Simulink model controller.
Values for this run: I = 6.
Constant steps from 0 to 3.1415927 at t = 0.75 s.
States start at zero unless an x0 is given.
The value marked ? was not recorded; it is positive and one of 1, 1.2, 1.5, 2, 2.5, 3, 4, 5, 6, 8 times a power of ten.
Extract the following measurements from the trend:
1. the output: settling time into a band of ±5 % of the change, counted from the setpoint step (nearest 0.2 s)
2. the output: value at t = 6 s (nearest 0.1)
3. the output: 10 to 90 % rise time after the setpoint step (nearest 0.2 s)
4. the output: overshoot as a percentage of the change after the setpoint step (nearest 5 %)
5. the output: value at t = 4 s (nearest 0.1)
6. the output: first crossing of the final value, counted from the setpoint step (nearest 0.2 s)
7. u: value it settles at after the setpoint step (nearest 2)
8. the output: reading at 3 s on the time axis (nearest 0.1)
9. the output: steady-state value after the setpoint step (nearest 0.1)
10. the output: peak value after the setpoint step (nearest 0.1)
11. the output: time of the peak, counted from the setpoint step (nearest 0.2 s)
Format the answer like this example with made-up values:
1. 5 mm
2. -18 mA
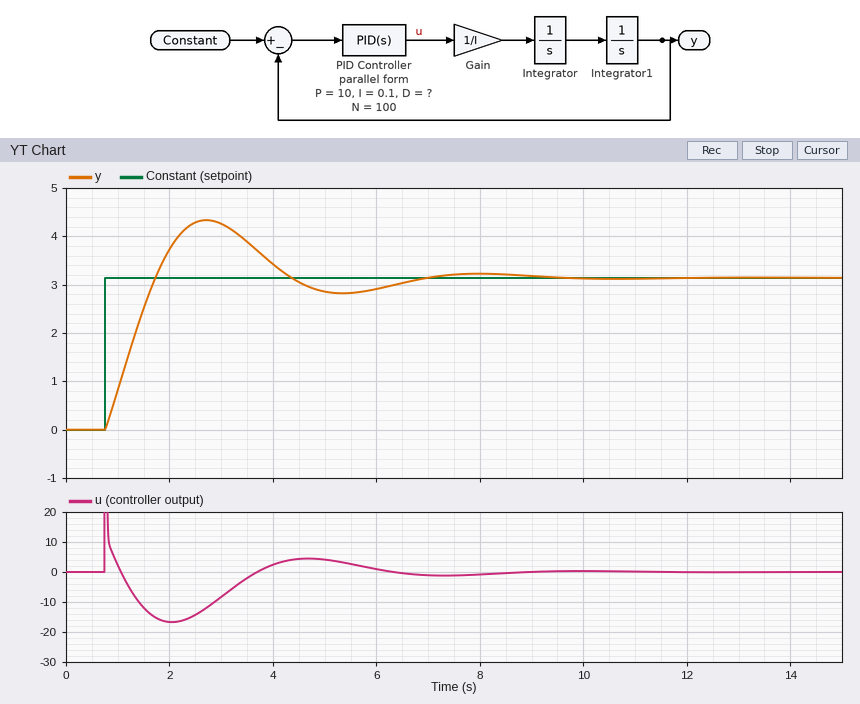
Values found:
1. 5.6 s
2. 2.9
3. 0.8 s
4. 40 %
5. 3.4
6. 1.0 s
7. 0
8. 4.3
9. 3.1
10. 4.3
11. 2.0 s
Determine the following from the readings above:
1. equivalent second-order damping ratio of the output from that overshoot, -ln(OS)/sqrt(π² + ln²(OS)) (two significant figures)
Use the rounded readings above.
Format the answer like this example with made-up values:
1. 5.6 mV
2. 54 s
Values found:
1. 0.28
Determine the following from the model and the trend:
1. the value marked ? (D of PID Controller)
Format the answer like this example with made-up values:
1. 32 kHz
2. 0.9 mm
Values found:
1. 6
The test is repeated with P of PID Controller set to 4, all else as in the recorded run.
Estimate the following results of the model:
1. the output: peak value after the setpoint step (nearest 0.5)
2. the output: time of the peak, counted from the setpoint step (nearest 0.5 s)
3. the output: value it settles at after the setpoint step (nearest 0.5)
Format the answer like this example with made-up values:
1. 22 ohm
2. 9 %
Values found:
1. 4.0
2. 3.0 s
3. 3.0
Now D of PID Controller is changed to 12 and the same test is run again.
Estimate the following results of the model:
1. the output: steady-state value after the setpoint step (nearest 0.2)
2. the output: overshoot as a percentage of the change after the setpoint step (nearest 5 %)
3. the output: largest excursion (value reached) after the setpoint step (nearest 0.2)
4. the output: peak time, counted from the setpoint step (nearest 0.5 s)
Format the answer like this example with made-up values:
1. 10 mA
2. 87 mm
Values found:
1. 3.2
2. 20 %
3. 3.8
4. 1.5 s
